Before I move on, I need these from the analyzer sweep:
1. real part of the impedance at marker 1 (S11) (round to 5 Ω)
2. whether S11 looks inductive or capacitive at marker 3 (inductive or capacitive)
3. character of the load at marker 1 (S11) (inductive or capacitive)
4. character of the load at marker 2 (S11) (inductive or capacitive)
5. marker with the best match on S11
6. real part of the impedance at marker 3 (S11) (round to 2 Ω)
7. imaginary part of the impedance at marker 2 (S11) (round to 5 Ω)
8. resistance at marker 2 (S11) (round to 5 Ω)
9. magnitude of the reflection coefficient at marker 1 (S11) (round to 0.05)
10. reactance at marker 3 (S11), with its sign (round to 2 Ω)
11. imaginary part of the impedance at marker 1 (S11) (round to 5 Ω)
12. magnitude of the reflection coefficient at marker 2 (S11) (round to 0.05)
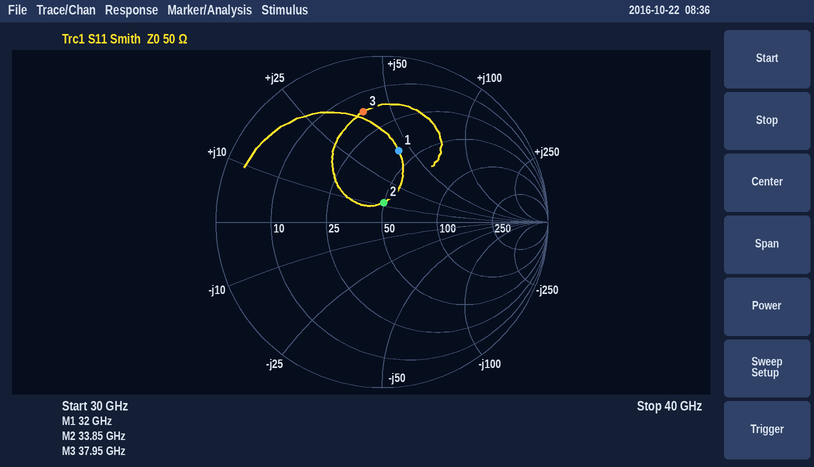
40 Ω
inductive
inductive
inductive
marker 2
16 Ω
+10 Ω
50 Ω
0.45
+40 Ω
+45 Ω
0.10
